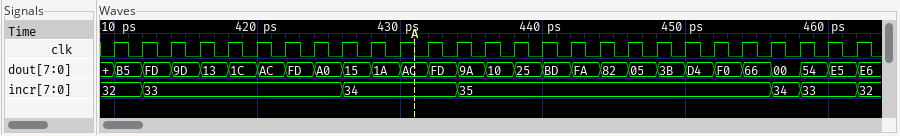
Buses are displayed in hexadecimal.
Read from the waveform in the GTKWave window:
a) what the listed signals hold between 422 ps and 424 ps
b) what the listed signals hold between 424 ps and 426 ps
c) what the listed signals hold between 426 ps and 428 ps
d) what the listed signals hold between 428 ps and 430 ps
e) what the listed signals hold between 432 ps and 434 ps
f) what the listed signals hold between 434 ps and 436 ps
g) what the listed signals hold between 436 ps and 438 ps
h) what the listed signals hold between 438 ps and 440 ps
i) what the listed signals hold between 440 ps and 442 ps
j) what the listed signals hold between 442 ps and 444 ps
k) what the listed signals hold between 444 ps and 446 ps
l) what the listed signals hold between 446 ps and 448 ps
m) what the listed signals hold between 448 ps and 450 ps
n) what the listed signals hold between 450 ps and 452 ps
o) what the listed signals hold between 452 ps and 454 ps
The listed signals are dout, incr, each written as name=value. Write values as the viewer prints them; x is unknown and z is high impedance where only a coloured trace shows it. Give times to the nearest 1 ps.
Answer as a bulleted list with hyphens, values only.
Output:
- dout=FD, incr=33
- dout=A0, incr=33
- dout=15, incr=34
- dout=1A, incr=34
- dout=FD, incr=34
- dout=9A, incr=35
- dout=10, incr=35
- dout=25, incr=35
- dout=BD, incr=35
- dout=FA, incr=35
- dout=82, incr=35
- dout=05, incr=35
- dout=3B, incr=35
- dout=D4, incr=35
- dout=F0, incr=35
